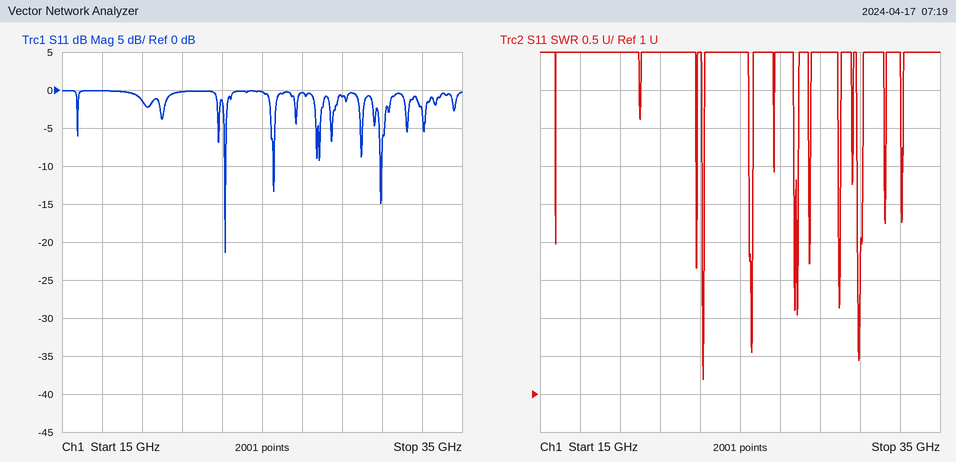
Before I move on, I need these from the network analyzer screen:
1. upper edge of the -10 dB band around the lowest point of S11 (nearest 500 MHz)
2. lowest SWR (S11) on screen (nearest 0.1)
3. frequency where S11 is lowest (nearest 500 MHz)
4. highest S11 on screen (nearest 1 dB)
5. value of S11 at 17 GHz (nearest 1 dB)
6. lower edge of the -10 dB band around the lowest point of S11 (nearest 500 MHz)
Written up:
23.0 GHz
1.2
23.0 GHz
0 dB
0 dB
23.0 GHz
